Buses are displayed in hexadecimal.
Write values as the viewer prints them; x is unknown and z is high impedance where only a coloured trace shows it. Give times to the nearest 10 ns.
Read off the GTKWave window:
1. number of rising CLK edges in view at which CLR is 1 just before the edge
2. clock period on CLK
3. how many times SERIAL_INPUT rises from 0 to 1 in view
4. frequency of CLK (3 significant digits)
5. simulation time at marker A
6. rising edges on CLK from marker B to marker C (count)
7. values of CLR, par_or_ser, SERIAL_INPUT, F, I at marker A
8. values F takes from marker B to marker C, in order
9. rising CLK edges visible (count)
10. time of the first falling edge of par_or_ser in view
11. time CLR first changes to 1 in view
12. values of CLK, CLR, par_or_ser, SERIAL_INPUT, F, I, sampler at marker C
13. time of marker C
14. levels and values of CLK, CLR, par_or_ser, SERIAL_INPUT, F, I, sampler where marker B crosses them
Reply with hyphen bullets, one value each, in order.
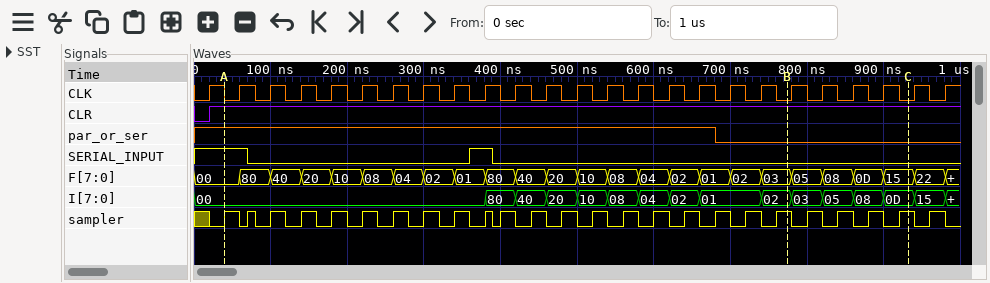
- 24
- 40 ns
- 1
- 25.0 MHz
- 40 ns
- 4
- CLR=1, par_or_ser=1, SERIAL_INPUT=1, F=00, I=00
- 03, 05, 08, 0D, 15
- 25
- 680 ns
- 20 ns
- CLK=0, CLR=1, par_or_ser=0, SERIAL_INPUT=0, F=15, I=0D, sampler=1
- 930 ns
- CLK=0, CLR=1, par_or_ser=0, SERIAL_INPUT=0, F=03, I=02, sampler=1
